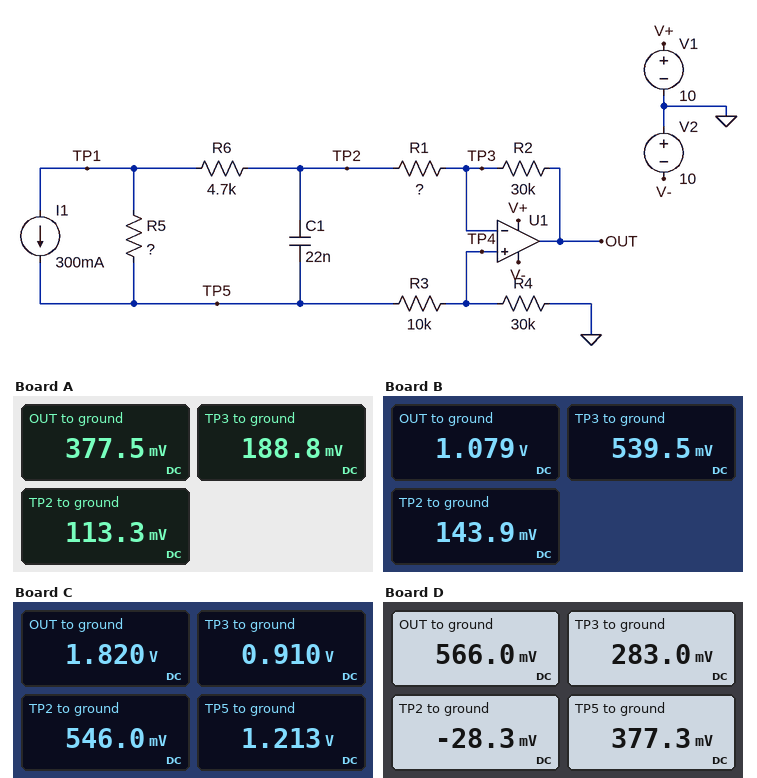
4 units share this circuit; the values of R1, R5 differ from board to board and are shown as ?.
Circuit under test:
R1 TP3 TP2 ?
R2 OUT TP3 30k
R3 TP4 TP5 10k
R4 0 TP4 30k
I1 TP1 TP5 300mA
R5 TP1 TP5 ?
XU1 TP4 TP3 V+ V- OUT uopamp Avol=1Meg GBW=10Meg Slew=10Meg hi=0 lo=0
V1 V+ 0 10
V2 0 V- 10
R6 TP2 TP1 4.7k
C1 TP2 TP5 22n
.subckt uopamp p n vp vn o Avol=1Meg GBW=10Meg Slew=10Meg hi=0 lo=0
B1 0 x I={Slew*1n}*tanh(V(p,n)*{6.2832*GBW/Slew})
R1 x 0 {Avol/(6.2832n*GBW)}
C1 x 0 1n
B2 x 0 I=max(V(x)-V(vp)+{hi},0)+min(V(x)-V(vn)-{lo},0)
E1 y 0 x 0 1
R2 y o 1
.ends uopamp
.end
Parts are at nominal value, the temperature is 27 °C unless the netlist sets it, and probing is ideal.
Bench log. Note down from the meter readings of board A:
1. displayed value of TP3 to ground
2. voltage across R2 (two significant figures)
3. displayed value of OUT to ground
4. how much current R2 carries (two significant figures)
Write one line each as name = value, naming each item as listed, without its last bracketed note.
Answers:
displayed value of TP3 to ground = 188.8 mV
voltage across R2 = 190 mV
displayed value of OUT to ground = 377.5 mV
how much current R2 carries = 6.3 µA
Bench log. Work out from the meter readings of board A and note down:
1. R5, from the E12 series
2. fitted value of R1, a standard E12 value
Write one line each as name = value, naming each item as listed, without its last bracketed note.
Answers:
R5, from the E12 series = 0.56 Ω
fitted value of R1, a standard E12 value = 12 kΩ
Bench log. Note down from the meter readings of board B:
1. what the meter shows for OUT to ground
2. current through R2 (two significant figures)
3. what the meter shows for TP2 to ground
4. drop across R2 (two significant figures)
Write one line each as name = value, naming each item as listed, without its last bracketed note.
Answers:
what the meter shows for OUT to ground = 1.079 V
current through R2 = 18 µA
what the meter shows for TP2 to ground = 143.9 mV
drop across R2 = 540 mV
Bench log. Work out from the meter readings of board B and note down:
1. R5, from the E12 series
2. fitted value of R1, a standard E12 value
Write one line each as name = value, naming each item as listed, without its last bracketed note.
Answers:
R5, from the E12 series = 2.2 Ω
fitted value of R1, a standard E12 value = 22 kΩ
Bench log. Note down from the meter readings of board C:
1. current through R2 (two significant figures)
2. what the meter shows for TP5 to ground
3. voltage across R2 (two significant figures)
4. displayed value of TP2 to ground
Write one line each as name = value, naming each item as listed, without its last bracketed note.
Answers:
current through R2 = 30 µA
what the meter shows for TP5 to ground = 1.213 V
voltage across R2 = 910 mV
displayed value of TP2 to ground = 546.0 mV
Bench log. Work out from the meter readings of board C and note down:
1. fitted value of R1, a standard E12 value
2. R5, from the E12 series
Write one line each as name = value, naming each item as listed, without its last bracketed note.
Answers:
fitted value of R1, a standard E12 value = 12 kΩ
R5, from the E12 series = 2.7 Ω
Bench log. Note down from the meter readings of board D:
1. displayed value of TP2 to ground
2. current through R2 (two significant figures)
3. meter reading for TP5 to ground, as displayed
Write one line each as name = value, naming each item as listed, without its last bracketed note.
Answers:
displayed value of TP2 to ground = -28.3 mV
current through R2 = 9.4 µA
meter reading for TP5 to ground, as displayed = 377.3 mV
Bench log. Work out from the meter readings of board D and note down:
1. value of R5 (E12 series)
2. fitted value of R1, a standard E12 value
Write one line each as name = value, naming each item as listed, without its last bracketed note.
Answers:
value of R5 = 1.5 Ω
fitted value of R1, a standard E12 value = 33 kΩ
